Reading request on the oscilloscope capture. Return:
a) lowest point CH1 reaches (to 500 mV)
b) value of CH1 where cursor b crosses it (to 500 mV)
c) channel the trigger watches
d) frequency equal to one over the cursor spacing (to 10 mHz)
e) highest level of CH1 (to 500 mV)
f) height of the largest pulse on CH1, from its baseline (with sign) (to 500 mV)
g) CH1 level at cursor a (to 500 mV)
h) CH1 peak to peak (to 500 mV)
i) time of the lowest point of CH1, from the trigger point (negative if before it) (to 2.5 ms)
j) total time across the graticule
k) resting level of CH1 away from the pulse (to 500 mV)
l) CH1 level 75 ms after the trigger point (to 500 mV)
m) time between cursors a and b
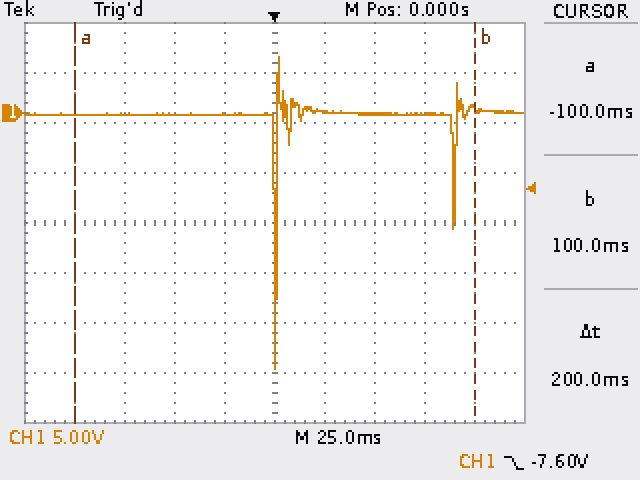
-25.5 V
500 mV
CH1
5.00 Hz
5.5 V
-25.5 V
0.0 V
31.0 V
0.0 ms
250 ms
0.0 V
0.0 V
200 ms
